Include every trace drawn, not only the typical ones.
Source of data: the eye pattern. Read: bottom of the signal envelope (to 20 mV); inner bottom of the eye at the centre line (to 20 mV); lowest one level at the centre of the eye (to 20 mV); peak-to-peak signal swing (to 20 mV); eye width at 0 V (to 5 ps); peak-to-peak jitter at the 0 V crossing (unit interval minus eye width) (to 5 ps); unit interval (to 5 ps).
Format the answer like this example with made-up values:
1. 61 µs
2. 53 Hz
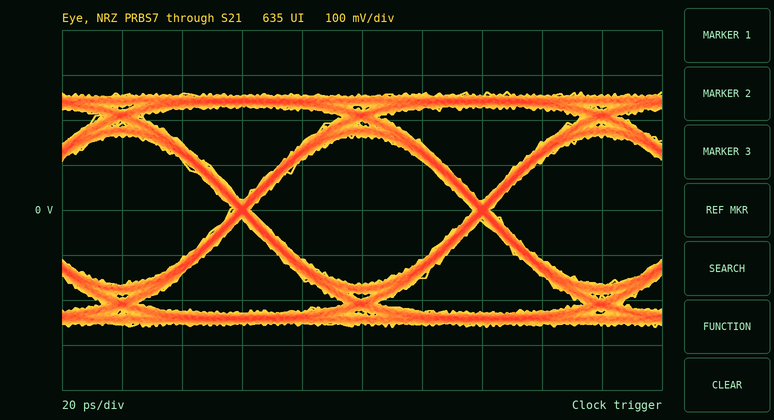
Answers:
1. -260 mV
2. -160 mV
3. 160 mV
4. 520 mV
5. 75 ps
6. 5 ps
7. 80 ps
